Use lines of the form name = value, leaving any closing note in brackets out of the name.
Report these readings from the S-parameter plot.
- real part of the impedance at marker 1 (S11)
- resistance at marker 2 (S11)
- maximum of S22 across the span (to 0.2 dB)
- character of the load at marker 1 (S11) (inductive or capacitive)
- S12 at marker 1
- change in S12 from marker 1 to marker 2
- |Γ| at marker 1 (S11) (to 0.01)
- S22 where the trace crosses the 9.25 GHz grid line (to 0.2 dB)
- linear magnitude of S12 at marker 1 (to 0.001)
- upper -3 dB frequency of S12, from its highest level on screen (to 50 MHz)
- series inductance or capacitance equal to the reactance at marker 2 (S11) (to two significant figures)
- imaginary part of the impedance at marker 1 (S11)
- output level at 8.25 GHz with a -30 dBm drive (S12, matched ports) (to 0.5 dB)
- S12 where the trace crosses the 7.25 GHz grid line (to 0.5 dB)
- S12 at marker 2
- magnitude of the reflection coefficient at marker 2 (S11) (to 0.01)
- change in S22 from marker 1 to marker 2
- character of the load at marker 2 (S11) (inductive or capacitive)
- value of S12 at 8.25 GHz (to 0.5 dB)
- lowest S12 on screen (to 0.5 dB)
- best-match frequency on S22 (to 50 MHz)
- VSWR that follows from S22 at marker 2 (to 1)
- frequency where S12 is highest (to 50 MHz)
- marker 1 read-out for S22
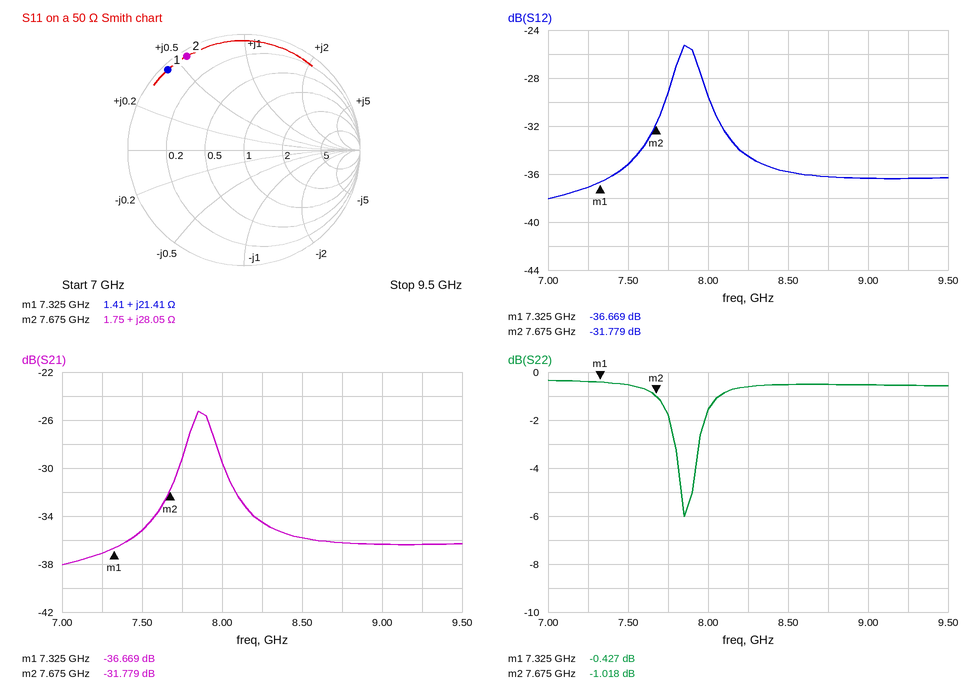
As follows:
real part of the impedance at marker 1 = 1.41 Ω
resistance at marker 2 = 1.75 Ω
maximum of S22 across the span = -0.4 dB
character of the load at marker 1 (S11) = inductive
S12 at marker 1 = -36.669 dB
change in S12 from marker 1 to marker 2 = 4.890 dB
|Γ| at marker 1 (S11) = 0.95
S22 where the trace crosses the 9.25 GHz grid line = -0.6 dB
linear magnitude of S12 at marker 1 = 0.015
upper -3 dB frequency of S12, from its highest level on screen = 7.95 GHz
series inductance or capacitance equal to the reactance at marker 2 (S11) = 580 pH
imaginary part of the impedance at marker 1 = +21.41 Ω
output level at 8.25 GHz with a -30 dBm drive (S12, matched ports) = -64.5 dBm
S12 where the trace crosses the 7.25 GHz grid line = -37.0 dB
S12 at marker 2 = -31.779 dB
magnitude of the reflection coefficient at marker 2 (S11) = 0.95
change in S22 from marker 1 to marker 2 = -0.591 dB
character of the load at marker 2 (S11) = inductive
value of S12 at 8.25 GHz = -34.5 dB
lowest S12 on screen = -38.0 dB
best-match frequency on S22 = 7.85 GHz
VSWR that follows from S22 at marker 2 = 17
frequency where S12 is highest = 7.85 GHz
marker 1 read-out for S22 = -0.427 dB
